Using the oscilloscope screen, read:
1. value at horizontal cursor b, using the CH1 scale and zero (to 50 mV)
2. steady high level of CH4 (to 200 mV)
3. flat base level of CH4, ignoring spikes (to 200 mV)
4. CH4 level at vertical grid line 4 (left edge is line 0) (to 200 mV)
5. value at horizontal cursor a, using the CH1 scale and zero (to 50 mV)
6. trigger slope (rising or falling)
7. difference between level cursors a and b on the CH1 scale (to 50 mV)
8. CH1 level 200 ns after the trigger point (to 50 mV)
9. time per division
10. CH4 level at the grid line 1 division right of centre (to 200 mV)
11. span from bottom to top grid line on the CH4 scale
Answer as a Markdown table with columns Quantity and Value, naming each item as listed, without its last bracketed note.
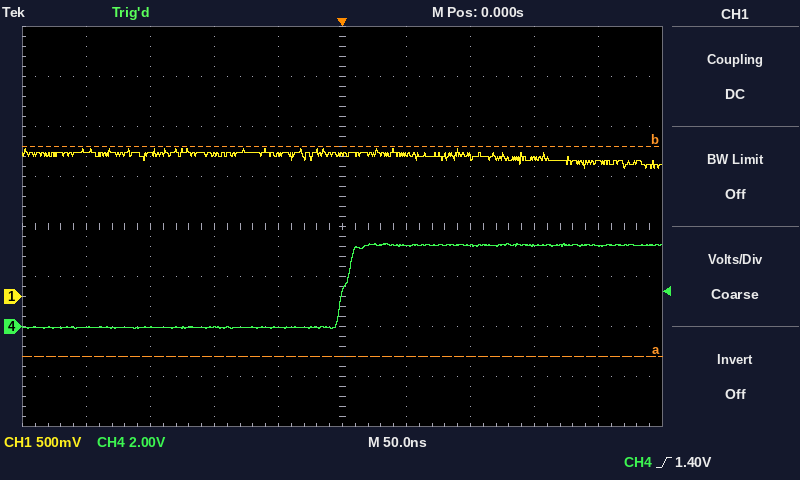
| Quantity | Value |
|---|---|
| value at horizontal cursor b, using the CH1 scale and zero | 1.50 V |
| steady high level of CH4 | 3.2 V |
| flat base level of CH4, ignoring spikes | 0.0 V |
| CH4 level at vertical grid line 4 (left edge is line 0) | 0.0 V |
| value at horizontal cursor a, using the CH1 scale and zero | -600 mV |
| trigger slope | rising |
| difference between level cursors a and b on the CH1 scale | 2.10 V |
| CH1 level 200 ns after the trigger point | 1.35 V |
| time per division | 50 ns |
| CH4 level at the grid line 1 division right of centre | 3.2 V |
| span from bottom to top grid line on the CH4 scale | 16 V |
